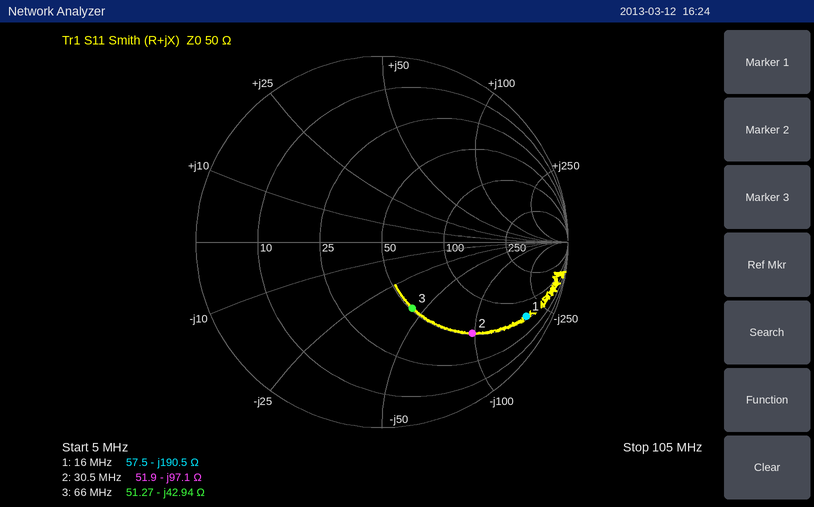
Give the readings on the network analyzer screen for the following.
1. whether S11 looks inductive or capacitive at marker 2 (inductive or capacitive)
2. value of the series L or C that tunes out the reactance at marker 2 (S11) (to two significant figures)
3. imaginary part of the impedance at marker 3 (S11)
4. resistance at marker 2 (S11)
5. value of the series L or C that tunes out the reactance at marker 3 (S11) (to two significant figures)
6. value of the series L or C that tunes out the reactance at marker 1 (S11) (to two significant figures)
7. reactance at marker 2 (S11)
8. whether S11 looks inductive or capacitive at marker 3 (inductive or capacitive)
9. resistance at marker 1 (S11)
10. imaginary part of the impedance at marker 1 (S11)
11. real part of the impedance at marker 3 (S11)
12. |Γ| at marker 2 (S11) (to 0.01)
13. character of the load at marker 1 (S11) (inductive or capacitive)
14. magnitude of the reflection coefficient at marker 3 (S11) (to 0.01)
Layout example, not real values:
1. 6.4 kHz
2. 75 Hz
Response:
1. capacitive
2. 510 nH
3. -42.94 Ω
4. 51.9 Ω
5. 100 nH
6. 1.9 µH
7. -97.1 Ω
8. capacitive
9. 57.5 Ω
10. -190.5 Ω
11. 51.27 Ω
12. 0.69
13. capacitive
14. 0.39
